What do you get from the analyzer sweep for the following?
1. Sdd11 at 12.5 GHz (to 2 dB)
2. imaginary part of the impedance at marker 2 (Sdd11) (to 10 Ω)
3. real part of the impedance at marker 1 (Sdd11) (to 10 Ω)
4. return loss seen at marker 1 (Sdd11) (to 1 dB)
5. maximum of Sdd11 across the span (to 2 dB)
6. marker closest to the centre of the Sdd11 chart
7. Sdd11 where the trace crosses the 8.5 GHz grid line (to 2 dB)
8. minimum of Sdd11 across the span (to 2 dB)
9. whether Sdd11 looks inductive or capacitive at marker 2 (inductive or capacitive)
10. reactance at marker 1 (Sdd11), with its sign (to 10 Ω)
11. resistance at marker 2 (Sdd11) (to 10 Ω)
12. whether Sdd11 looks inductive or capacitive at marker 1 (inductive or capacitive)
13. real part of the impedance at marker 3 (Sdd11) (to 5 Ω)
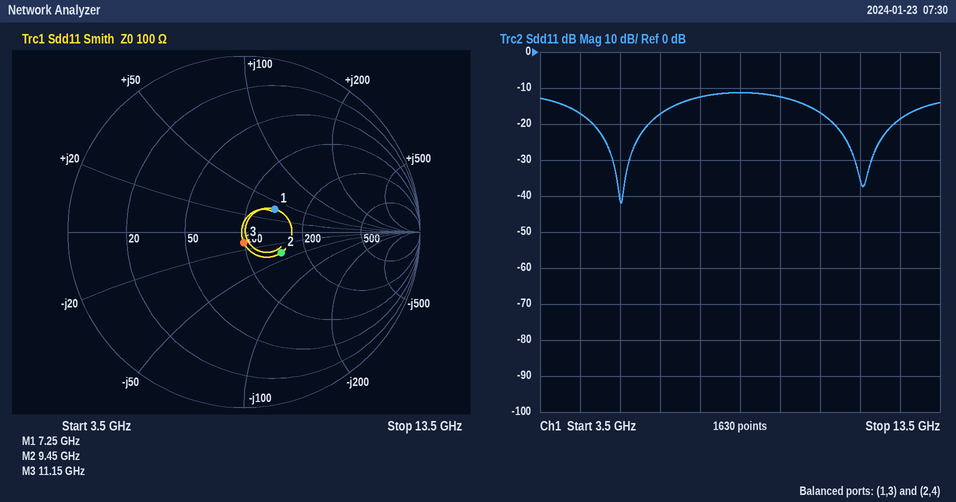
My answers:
-18 dB
-40 Ω
140 Ω
13 dB
-12 dB
marker 3
-12 dB
-42 dB
capacitive
+40 Ω
150 Ω
inductive
100 Ω
